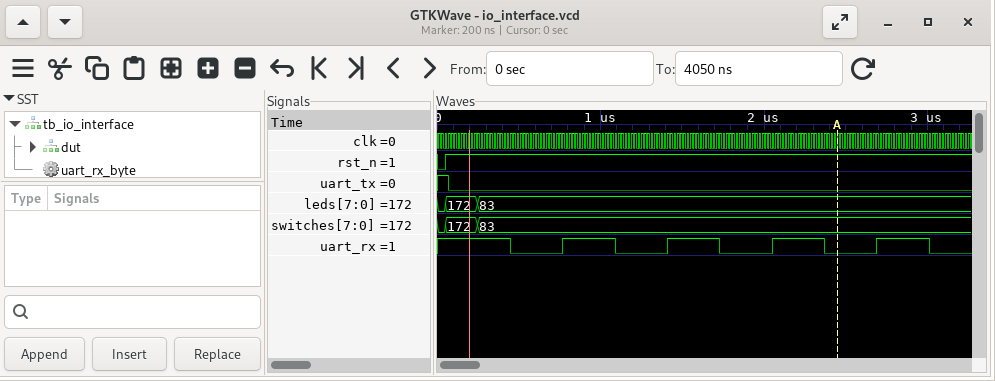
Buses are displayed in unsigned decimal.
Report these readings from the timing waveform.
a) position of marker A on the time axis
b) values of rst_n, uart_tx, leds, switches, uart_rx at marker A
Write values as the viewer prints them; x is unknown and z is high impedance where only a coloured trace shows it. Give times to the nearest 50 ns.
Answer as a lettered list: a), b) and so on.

a) 2450 ns
b) rst_n=1, uart_tx=0, leds=83, switches=83, uart_rx=0
